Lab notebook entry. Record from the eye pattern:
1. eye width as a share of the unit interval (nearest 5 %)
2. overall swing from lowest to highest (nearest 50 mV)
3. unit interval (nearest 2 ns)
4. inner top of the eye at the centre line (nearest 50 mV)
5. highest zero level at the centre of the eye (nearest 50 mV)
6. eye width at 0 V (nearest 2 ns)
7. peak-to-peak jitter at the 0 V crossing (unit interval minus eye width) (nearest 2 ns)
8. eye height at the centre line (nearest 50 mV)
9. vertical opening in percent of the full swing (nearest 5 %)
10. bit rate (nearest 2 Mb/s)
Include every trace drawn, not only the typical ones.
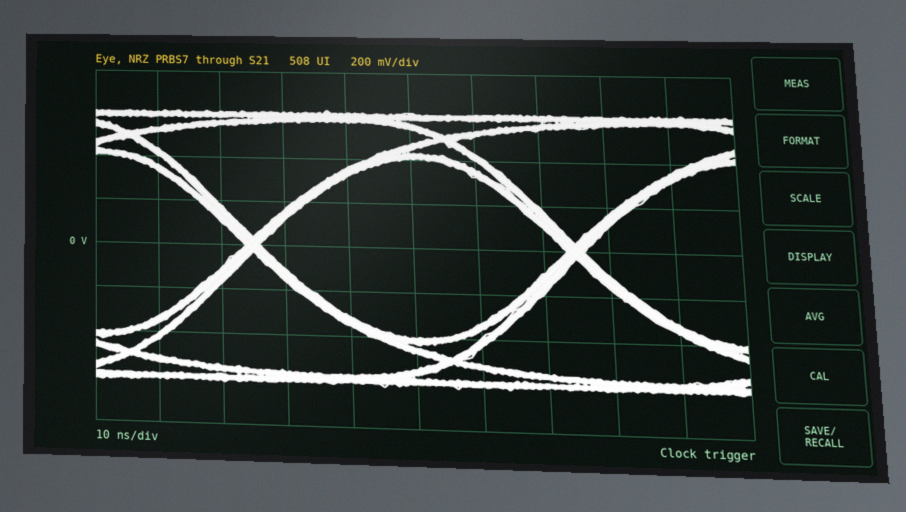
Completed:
95 %
1.25 V
50 ns
400 mV
-400 mV
48 ns
2 ns
800 mV
65 %
20 Mb/s
